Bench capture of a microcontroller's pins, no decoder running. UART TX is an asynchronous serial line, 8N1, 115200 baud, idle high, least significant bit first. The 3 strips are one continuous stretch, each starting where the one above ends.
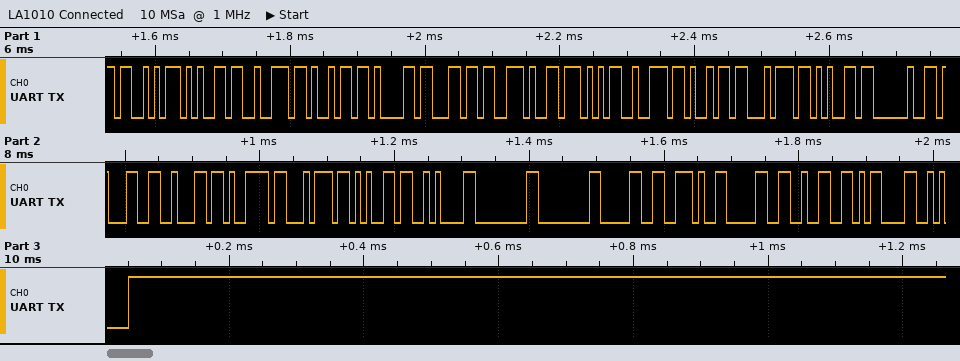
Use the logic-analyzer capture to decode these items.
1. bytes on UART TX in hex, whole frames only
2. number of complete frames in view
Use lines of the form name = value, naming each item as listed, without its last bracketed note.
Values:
bytes on UART TX in hex, whole frames only = 53 65 72 69 61 6C 2E 57 72 69 74 65 20 31 62 79 74 65 0A 00 00 30 2E 30 32 0D 0A
number of complete frames in view = 27
